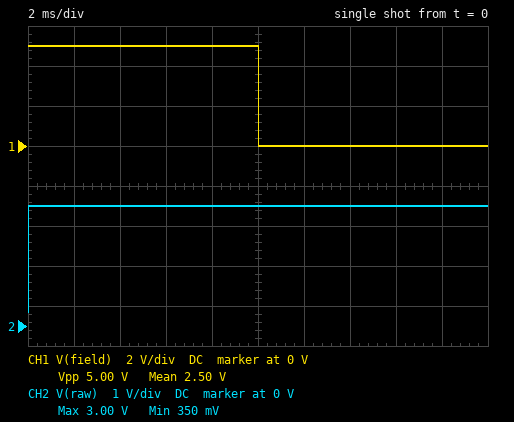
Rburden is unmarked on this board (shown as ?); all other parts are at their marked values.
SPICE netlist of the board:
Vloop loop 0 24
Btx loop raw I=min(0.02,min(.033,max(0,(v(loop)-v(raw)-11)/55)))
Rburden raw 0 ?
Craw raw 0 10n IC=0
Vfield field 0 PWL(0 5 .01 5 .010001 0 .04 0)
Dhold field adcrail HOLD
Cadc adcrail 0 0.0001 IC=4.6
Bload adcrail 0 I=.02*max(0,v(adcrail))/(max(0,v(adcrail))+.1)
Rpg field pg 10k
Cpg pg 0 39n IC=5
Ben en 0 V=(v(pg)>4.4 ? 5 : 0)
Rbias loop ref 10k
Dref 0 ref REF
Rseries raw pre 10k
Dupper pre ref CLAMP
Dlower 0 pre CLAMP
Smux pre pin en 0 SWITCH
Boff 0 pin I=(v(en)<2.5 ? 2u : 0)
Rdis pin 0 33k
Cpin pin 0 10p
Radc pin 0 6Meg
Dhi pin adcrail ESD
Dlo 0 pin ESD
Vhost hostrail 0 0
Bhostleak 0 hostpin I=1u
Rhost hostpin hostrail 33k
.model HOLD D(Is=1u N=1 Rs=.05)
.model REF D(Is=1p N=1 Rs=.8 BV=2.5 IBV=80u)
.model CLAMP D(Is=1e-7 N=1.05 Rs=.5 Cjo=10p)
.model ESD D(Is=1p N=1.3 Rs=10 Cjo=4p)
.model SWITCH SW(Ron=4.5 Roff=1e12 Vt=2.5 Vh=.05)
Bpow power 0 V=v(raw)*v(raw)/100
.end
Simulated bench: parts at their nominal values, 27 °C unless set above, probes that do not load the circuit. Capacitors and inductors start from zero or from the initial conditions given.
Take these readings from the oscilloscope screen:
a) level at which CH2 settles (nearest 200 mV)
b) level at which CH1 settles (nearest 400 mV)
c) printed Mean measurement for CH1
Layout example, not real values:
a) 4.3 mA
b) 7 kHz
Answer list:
a) 3.0 V
b) 0 V
c) 2.50 V
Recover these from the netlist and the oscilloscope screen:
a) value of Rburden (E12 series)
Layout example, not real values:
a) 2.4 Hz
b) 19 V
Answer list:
a) 150 Ω
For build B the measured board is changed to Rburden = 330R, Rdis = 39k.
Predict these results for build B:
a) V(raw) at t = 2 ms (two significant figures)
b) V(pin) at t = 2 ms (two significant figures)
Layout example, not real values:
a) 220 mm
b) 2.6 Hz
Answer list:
a) 6.5 V
b) 2.8 V
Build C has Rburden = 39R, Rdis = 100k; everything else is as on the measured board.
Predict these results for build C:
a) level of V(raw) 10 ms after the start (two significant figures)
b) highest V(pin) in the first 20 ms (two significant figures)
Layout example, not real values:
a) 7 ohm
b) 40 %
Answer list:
a) 780 mV
b) 710 mV
